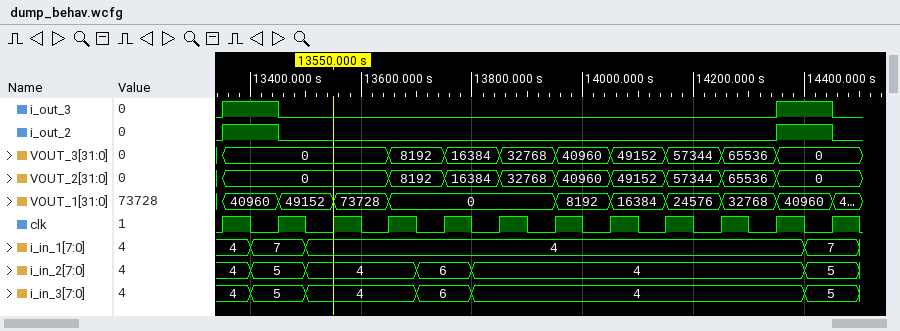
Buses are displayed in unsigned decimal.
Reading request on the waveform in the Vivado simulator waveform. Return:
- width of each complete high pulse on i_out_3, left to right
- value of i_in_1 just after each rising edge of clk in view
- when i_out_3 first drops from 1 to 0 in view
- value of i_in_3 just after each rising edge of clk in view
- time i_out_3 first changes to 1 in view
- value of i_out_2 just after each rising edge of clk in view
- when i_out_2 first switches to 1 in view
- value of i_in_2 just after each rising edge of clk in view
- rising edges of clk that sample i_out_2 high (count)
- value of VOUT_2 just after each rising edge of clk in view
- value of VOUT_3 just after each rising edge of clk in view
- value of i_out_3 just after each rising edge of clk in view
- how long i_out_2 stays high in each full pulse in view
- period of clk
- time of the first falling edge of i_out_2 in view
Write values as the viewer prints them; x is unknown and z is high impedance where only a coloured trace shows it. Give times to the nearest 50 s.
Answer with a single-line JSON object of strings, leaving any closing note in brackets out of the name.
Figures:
{"width of each complete high pulse on i_out_3, left to right": "100 s, 100 s", "value of i_in_1 just after each rising edge of clk in view": "4, 7, 4, 4, 4, 4, 4, 4, 4, 4, 4, 7", "when i_out_3 first drops from 1 to 0 in view": "13450 s", "value of i_in_3 just after each rising edge of clk in view": "4, 5, 4, 4, 6, 4, 4, 4, 4, 4, 4, 5", "time i_out_3 first changes to 1 in view": "13350 s", "value of i_out_2 just after each rising edge of clk in view": "1 0 0 0 0 0 0 0 0 0 1 0", "when i_out_2 first switches to 1 in view": "13350 s", "value of i_in_2 just after each rising edge of clk in view": "4, 5, 4, 4, 6, 4, 4, 4, 4, 4, 4, 5", "rising edges of clk that sample i_out_2 high": "2", "value of VOUT_2 just after each rising edge of clk in view": "0, 0, 0, 8192, 16384, 32768, 40960, 49152, 57344, 65536, 0, 0", "value of VOUT_3 just after each rising edge of clk in view": "0, 0, 0, 8192, 16384, 32768, 40960, 49152, 57344, 65536, 0, 0", "value of i_out_3 just after each rising edge of clk in view": "1 0 0 0 0 0 0 0 0 0 1 0", "how long i_out_2 stays high in each full pulse in view": "100 s, 100 s", "period of clk": "100 s", "time of the first falling edge of i_out_2 in view": "13450 s"}
